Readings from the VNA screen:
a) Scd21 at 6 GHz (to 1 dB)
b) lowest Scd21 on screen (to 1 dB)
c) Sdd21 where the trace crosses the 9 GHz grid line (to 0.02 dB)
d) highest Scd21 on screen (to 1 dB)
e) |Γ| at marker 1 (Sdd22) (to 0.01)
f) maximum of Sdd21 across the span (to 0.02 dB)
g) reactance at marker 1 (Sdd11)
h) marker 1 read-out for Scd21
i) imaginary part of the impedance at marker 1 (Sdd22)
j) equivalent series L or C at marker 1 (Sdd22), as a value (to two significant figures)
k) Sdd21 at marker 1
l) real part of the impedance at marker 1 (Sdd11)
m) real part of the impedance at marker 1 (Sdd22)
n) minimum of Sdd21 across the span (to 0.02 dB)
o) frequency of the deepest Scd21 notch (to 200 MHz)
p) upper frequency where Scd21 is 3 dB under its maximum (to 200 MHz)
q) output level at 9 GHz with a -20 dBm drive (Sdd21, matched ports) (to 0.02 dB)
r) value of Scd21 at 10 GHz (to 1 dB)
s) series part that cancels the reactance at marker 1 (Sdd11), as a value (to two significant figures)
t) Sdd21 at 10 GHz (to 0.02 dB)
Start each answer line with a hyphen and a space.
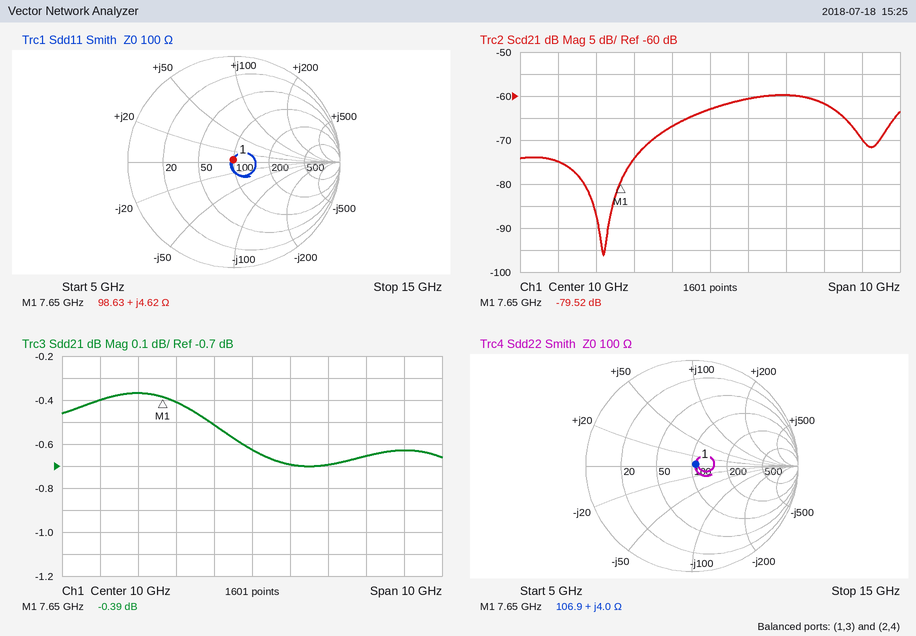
- -75 dB
- -96 dB
- -0.52 dB
- -60 dB
- 0.04
- -0.36 dB
- +4.62 Ω
- -79.52 dB
- +4.0 Ω
- 83 pH
- -0.39 dB
- 98.63 Ω
- 106.9 Ω
- -0.70 dB
- 7.2 GHz
- 13.2 GHz
- -20.52 dBm
- -63 dB
- 4.5 pF
- -0.62 dB
